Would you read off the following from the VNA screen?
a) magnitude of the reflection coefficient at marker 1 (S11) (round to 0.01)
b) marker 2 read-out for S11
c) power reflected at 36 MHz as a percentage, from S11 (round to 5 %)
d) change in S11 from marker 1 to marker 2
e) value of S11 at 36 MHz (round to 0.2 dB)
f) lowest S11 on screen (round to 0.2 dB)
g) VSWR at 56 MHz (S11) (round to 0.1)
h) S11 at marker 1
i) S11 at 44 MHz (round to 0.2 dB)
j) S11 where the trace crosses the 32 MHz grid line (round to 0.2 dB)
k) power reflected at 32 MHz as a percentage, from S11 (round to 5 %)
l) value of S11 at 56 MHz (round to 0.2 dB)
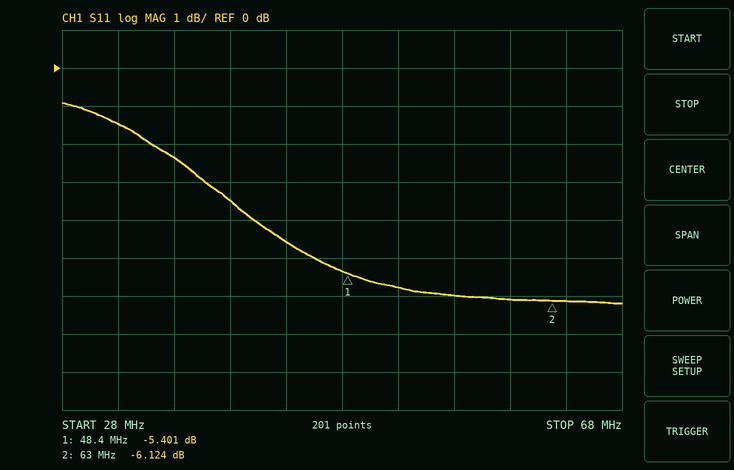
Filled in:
0.54
-6.124 dB
60 %
-0.723 dB
-2.4 dB
-6.2 dB
3.0
-5.401 dB
-4.6 dB
-1.4 dB
70 %
-6.0 dB
